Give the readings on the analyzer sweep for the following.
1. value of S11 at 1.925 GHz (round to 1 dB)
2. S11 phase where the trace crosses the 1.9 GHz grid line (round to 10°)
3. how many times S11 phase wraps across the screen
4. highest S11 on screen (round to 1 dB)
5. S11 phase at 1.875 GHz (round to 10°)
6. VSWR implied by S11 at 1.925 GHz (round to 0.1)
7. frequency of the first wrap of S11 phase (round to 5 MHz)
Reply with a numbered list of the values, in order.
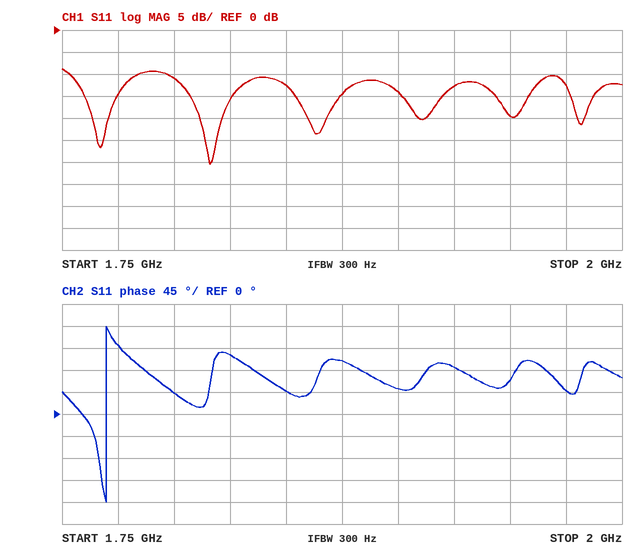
1. -13 dB
2. 50°
3. 1
4. -9 dB
5. 110°
6. 1.6
7. 1.770 GHz
